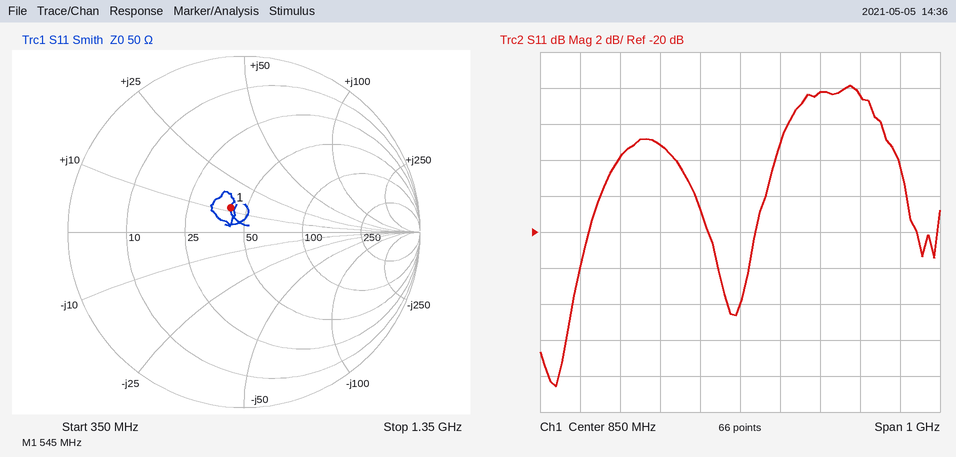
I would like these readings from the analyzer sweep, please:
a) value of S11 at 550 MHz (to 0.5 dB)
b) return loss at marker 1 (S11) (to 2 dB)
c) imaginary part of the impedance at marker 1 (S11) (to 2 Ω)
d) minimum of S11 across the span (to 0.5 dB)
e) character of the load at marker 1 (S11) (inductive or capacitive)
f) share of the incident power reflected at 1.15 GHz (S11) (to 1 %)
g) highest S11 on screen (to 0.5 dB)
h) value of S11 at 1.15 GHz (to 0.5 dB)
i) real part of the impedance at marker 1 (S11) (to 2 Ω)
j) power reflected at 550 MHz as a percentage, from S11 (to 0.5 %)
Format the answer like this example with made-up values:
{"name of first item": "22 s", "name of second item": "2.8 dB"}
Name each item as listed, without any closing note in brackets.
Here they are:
{"value of S11 at 550 MHz": "-16.0 dB", "return loss at marker 1 (S11)": "16 dB", "imaginary part of the impedance at marker 1 (S11)": "+12 Ω", "minimum of S11 across the span": "-28.5 dB", "character of the load at marker 1 (S11)": "inductive", "share of the incident power reflected at 1.15 GHz (S11)": "6 %", "highest S11 on screen": "-12.0 dB", "value of S11 at 1.15 GHz": "-12.5 dB", "real part of the impedance at marker 1 (S11)": "42 Ω", "power reflected at 550 MHz as a percentage, from S11": "2.5 %"}
